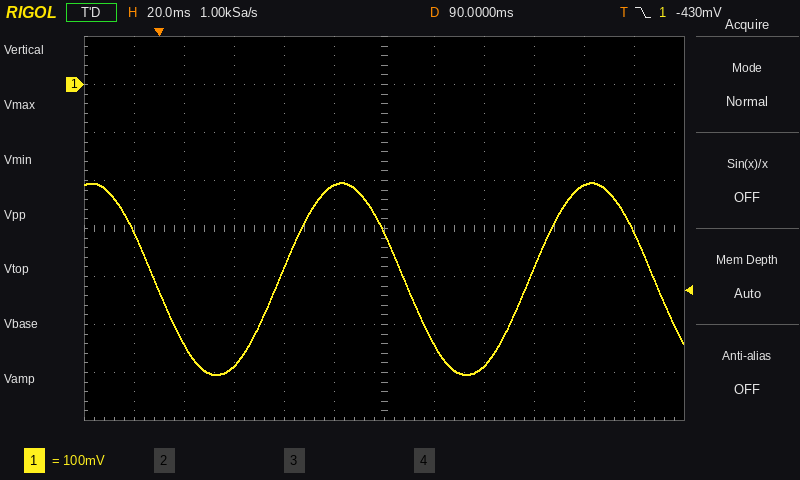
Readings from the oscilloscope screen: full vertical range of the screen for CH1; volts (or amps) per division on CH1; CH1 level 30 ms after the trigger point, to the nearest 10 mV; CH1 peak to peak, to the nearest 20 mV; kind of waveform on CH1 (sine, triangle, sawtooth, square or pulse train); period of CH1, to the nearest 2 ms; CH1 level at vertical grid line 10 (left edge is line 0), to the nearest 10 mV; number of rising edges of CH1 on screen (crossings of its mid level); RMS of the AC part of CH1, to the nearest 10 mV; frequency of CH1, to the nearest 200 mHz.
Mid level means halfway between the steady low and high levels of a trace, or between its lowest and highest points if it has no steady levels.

800 mV
100 mV
-590 mV
400 mV
sine
100 ms
-210 mV
2
140 mV
10.0 Hz
